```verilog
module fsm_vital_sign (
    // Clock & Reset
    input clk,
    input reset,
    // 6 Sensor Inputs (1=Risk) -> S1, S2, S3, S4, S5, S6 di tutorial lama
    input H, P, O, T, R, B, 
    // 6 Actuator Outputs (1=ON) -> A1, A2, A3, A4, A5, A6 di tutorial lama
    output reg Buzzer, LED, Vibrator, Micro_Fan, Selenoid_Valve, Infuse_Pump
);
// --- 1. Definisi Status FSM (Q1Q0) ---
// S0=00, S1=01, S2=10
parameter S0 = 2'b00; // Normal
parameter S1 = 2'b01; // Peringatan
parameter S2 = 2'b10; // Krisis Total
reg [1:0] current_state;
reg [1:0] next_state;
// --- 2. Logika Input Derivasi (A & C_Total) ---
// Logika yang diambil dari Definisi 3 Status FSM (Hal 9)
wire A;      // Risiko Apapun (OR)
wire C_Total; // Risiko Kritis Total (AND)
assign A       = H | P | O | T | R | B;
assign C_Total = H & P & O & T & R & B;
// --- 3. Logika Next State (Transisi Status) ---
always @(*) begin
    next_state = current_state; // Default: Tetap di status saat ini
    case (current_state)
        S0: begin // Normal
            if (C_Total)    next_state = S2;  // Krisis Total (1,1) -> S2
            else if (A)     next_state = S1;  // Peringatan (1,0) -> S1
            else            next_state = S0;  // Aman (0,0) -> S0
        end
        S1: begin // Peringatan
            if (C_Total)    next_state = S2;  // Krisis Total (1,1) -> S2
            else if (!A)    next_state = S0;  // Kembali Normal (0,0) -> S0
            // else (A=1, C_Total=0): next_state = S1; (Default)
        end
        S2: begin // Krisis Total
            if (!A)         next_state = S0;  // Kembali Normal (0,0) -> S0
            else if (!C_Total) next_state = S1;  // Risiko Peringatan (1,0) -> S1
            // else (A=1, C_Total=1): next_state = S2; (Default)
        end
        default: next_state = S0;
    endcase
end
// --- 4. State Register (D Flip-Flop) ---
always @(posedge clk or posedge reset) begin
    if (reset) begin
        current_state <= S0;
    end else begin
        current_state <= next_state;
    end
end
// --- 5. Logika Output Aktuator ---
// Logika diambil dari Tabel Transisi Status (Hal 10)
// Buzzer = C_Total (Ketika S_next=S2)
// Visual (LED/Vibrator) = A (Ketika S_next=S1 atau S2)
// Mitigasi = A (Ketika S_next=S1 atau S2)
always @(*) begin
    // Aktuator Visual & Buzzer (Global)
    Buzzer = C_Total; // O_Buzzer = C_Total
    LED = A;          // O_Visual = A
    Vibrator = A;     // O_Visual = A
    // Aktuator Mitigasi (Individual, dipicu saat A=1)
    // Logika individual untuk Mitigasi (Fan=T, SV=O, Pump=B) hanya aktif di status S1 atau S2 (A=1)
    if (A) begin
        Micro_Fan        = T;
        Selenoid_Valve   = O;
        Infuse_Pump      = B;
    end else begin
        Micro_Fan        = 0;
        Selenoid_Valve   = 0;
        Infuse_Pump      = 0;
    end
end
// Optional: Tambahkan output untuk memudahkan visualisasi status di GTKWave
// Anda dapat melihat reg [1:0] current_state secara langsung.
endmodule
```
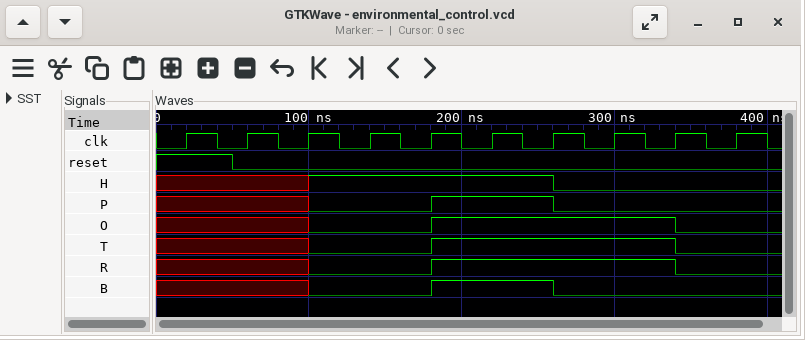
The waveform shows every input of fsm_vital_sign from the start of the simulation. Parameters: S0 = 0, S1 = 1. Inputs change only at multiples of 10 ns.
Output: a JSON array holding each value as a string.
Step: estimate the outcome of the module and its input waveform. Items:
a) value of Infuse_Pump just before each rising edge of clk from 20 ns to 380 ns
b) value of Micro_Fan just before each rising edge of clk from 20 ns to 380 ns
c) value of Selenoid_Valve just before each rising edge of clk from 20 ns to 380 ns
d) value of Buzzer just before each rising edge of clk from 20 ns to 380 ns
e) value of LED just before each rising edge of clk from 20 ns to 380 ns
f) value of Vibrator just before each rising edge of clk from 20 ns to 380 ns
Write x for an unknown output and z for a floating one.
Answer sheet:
["x x x 0 0 1 1 0 0 0", "x x x 0 0 1 1 1 1 0", "x x x 0 0 1 1 1 1 0", "x x x 0 0 1 1 0 0 0", "x x x 1 1 1 1 1 1 0", "x x x 1 1 1 1 1 1 0"]
